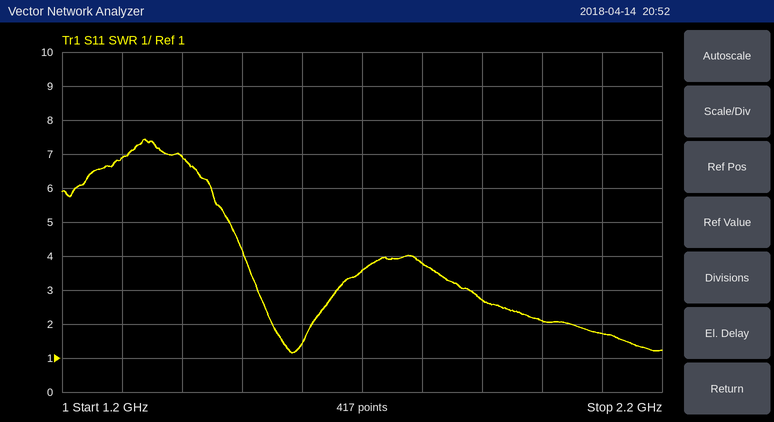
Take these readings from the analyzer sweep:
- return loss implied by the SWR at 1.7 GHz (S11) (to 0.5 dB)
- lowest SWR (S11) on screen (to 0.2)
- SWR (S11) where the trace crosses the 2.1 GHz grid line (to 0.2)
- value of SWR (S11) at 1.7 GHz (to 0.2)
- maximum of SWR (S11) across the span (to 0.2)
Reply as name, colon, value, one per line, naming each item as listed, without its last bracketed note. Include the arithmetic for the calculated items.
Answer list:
return loss implied by the SWR at 1.7 GHz (S11): −20 log10((3.6 − 1)/(3.6 + 1)) ≈ 5.0 dB
lowest SWR (S11) on screen: 1.2
SWR (S11) where the trace crosses the 2.1 GHz grid line: 1.8
value of SWR (S11) at 1.7 GHz: 3.6
maximum of SWR (S11) across the span: 7.4
